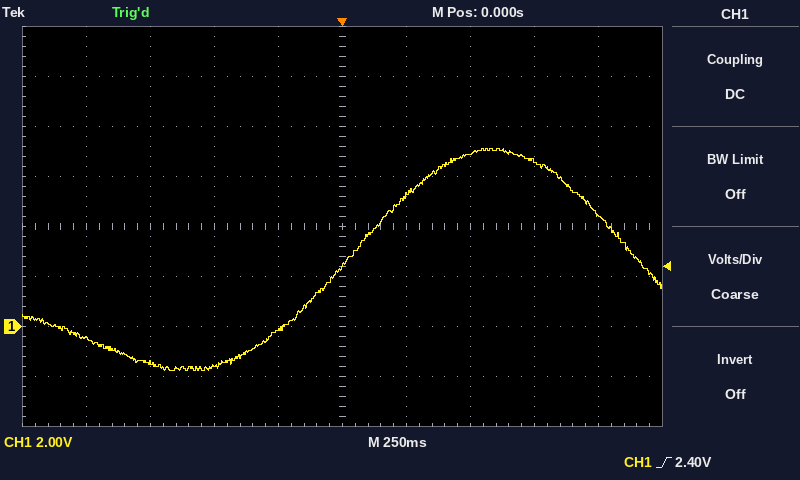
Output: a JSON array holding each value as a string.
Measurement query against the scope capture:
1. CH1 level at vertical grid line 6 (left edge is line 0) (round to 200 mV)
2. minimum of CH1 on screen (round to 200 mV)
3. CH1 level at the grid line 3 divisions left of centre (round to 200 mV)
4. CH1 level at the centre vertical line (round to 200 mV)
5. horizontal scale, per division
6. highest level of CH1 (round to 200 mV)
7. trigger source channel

["5.2 V", "-1.8 V", "-1.4 V", "2.4 V", "250 ms", "7.2 V", "CH1"]
